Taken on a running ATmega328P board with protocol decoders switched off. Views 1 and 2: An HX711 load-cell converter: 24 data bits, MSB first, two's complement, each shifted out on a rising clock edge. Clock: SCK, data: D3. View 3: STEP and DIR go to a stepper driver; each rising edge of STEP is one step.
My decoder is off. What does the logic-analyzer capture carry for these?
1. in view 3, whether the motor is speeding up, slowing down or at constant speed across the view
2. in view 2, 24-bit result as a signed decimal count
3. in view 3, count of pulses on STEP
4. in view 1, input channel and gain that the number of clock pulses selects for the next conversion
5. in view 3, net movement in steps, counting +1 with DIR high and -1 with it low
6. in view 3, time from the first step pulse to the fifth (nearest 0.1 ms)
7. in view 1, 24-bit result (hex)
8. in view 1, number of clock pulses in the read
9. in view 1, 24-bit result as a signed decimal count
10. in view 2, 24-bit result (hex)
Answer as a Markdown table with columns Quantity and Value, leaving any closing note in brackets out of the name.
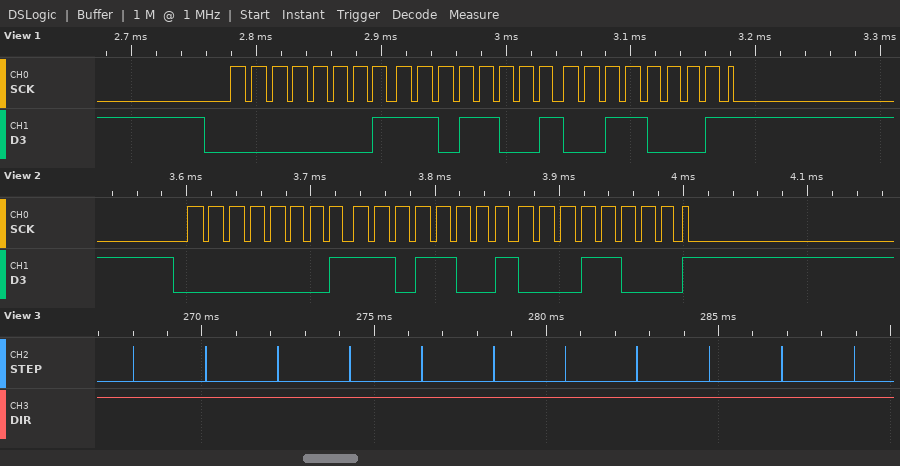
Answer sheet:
| Quantity | Value |
|---|---|
| in view 3, whether the motor is speeding up, slowing down or at constant speed across the view | constant speed |
| in view 2, 24-bit result as a signed decimal count | 121112 |
| in view 3, count of pulses on STEP | 11 |
| in view 1, input channel and gain that the number of clock pulses selects for the next conversion | channel A, gain 128 |
| in view 3, net movement in steps, counting +1 with DIR high and -1 with it low | +11 |
| in view 3, time from the first step pulse to the fifth | 8.4 ms |
| in view 1, 24-bit result | 0x01D931 |
| in view 1, number of clock pulses in the read | 25 |
| in view 1, 24-bit result as a signed decimal count | 121137 |
| in view 2, 24-bit result | 0x01D918 |
